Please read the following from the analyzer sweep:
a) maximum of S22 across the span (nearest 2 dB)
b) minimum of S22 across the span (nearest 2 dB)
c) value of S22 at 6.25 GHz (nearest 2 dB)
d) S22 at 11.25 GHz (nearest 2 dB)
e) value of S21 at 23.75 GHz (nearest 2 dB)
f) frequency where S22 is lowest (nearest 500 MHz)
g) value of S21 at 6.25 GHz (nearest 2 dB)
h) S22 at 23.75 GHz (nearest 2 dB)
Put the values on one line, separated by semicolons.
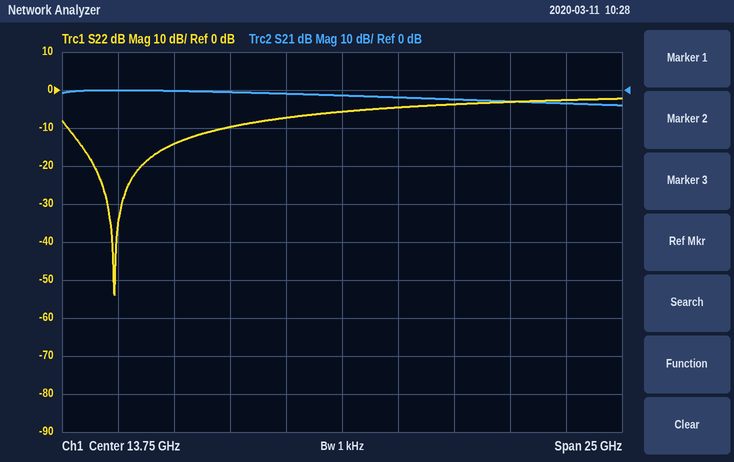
-2 dB; -54 dB; -14 dB; -8 dB; -4 dB; 3.5 GHz; 0 dB; -2 dB
